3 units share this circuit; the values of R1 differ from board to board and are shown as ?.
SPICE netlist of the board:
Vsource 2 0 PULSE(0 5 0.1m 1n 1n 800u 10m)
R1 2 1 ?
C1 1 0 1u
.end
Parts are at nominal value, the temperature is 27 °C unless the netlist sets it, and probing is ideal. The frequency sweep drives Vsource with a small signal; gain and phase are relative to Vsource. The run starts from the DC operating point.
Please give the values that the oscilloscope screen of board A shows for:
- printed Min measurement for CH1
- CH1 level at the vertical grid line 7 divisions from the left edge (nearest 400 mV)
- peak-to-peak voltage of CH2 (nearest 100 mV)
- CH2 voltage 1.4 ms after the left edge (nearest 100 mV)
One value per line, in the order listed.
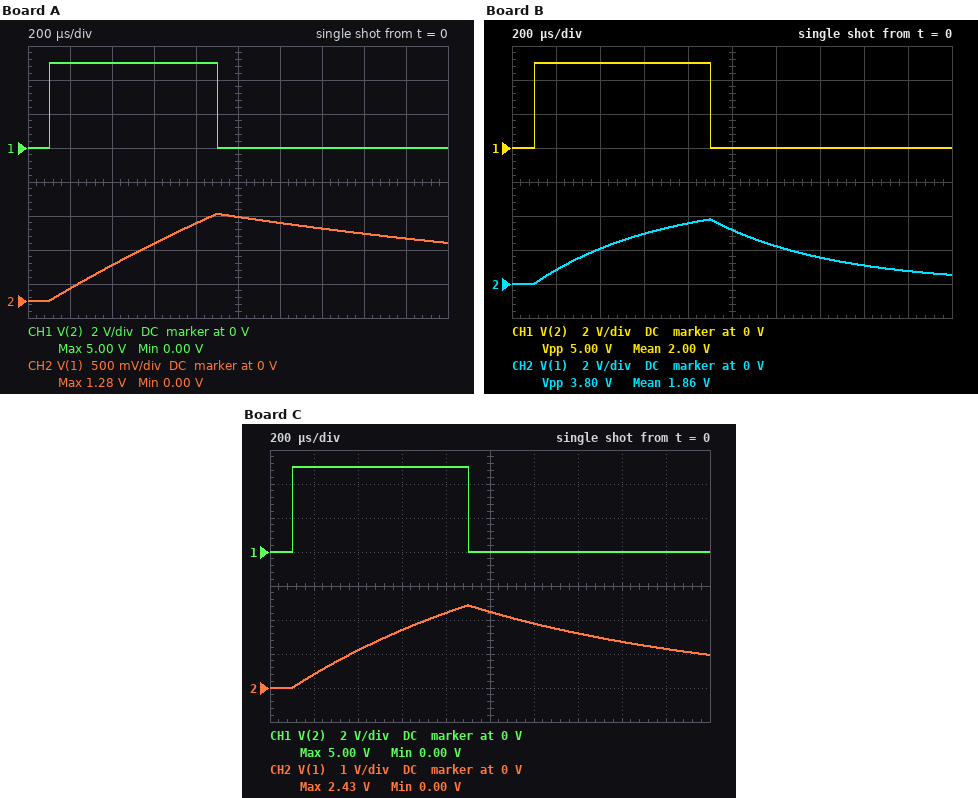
0.00 V
0 V
1.3 V
1.1 V
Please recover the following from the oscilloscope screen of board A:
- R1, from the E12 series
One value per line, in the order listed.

2.7 kΩ
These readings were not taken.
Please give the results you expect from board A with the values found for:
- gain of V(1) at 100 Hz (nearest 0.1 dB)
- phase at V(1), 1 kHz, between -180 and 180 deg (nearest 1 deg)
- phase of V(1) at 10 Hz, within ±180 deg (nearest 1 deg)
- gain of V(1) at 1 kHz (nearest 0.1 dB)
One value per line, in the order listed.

-5.9 dB
-87 deg
-10 deg
-24.6 dB
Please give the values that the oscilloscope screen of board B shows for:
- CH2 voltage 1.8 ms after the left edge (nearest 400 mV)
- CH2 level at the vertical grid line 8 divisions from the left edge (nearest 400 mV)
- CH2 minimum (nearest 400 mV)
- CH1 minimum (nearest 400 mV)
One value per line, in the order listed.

800 mV
1.2 V
0 V
0 V
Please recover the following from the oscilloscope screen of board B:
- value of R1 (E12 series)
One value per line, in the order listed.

560 Ω
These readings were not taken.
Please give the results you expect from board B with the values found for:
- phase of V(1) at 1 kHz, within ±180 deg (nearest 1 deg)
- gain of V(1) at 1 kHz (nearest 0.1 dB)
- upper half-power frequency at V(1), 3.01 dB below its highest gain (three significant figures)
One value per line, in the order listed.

-74 deg
-11.3 dB
284 Hz
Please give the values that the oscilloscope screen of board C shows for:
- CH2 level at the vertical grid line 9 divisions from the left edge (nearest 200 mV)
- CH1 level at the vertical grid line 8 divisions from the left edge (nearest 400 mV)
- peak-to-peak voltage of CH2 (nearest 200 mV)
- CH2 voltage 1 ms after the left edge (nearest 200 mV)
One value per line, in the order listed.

1.2 V
0 V
2.4 V
2.2 V
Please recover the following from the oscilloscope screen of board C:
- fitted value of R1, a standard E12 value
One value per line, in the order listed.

1.2 kΩ
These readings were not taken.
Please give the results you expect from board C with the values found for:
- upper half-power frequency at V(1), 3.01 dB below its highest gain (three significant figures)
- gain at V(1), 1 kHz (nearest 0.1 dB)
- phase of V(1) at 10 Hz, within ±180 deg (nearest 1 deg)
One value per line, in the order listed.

133 Hz
-17.6 dB
-4 deg
